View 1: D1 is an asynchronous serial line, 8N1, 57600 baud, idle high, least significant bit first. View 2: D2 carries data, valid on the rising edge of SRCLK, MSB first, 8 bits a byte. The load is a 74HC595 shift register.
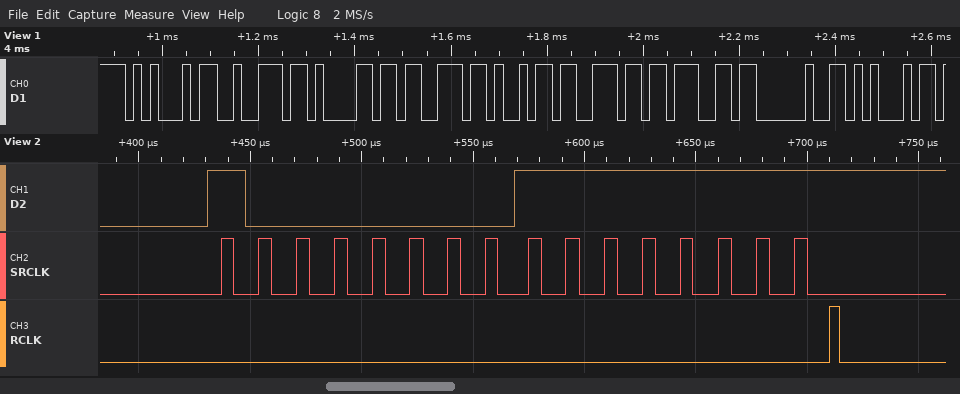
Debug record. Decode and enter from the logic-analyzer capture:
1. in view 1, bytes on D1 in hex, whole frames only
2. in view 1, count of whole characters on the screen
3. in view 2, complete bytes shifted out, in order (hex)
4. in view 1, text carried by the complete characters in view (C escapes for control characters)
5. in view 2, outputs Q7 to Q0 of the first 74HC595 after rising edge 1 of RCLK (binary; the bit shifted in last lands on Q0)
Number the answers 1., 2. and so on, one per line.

1. 45 72 61 73 69 6E 67 20 45
2. 9
3. 80 FF
4. "Erasing E"
5. 11111111
